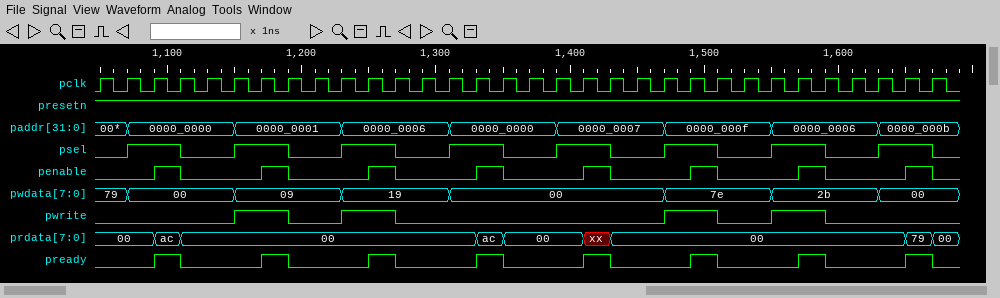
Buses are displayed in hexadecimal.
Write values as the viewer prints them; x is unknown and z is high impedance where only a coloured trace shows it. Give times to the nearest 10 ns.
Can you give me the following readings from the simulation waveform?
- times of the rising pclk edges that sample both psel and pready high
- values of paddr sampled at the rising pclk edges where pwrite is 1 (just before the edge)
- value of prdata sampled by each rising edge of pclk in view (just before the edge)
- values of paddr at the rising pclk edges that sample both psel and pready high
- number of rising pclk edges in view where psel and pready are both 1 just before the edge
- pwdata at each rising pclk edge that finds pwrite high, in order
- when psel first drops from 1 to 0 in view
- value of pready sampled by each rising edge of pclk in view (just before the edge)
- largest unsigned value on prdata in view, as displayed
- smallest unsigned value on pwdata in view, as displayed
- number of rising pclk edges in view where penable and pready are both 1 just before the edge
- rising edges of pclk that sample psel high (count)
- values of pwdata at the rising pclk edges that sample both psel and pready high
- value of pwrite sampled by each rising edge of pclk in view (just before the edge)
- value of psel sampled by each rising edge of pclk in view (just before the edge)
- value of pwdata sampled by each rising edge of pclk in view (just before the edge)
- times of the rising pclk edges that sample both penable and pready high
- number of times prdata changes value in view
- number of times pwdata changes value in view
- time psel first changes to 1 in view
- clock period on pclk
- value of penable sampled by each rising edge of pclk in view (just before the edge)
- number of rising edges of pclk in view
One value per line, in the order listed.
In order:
1110 ns, 1190 ns, 1270 ns, 1350 ns, 1430 ns, 1510 ns, 1590 ns, 1670 ns
0000_0001, 0000_0001, 0000_0006, 0000_0006, 0000_000f, 0000_000f, 0000_0006, 0000_0006
00, 00, 00, ac, 00, 00, 00, 00, 00, 00, 00, 00, 00, 00, 00, ac, 00, 00, 00, xx, 00, 00, 00, 00, 00, 00, 00, 00, 00, 00, 00, 79
0000_0000, 0000_0001, 0000_0006, 0000_0000, 0000_0007, 0000_000f, 0000_0006, 0000_000b
8
09, 09, 19, 19, 7e, 7e, 2b, 2b
1110 ns
0 0 0 1 0 0 0 1 0 0 0 1 0 0 0 1 0 0 0 1 0 0 0 1 0 0 0 1 0 0 0 1
ac
00
8
16
00, 09, 19, 00, 00, 7e, 2b, 00
0 0 0 0 0 0 1 1 0 0 1 1 0 0 0 0 0 0 0 0 0 0 1 1 0 0 1 1 0 0 0 0
0 0 1 1 0 0 1 1 0 0 1 1 0 0 1 1 0 0 1 1 0 0 1 1 0 0 1 1 0 0 1 1
79, 79, 00, 00, 00, 00, 09, 09, 09, 09, 19, 19, 19, 19, 00, 00, 00, 00, 00, 00, 00, 00, 7e, 7e, 7e, 7e, 2b, 2b, 2b, 2b, 00, 00
1110 ns, 1190 ns, 1270 ns, 1350 ns, 1430 ns, 1510 ns, 1590 ns, 1670 ns
8
7
1070 ns
20 ns
0 0 0 1 0 0 0 1 0 0 0 1 0 0 0 1 0 0 0 1 0 0 0 1 0 0 0 1 0 0 0 1
32
